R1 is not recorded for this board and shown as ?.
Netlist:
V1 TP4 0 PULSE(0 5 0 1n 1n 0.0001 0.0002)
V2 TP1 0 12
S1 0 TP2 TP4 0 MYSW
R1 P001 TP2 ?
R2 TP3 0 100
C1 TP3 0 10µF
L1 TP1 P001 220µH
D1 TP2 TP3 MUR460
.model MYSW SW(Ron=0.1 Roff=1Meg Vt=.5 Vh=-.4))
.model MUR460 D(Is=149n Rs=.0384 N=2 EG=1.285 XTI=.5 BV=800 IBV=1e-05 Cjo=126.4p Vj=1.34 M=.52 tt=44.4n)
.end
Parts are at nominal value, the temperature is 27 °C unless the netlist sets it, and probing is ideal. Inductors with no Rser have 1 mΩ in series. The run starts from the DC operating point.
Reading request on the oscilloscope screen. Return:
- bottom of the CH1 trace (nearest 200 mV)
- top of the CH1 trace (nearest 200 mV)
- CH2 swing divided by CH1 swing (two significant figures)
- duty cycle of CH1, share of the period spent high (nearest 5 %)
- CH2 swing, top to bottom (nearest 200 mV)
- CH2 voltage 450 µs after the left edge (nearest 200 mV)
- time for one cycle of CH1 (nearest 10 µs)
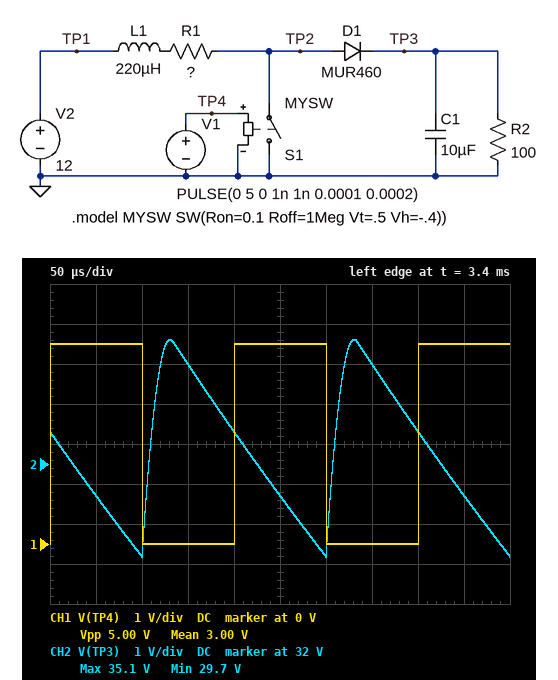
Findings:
0 V
5.0 V
1.1
50 %
5.4 V
31.2 V
200 µs
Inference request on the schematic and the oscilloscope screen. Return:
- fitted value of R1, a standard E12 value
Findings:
1.5 Ω
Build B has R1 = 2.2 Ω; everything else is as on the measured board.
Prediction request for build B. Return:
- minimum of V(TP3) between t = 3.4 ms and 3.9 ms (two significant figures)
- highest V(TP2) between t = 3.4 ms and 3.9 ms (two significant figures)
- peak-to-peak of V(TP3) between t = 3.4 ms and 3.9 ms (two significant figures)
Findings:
26 V
31 V
4.7 V
